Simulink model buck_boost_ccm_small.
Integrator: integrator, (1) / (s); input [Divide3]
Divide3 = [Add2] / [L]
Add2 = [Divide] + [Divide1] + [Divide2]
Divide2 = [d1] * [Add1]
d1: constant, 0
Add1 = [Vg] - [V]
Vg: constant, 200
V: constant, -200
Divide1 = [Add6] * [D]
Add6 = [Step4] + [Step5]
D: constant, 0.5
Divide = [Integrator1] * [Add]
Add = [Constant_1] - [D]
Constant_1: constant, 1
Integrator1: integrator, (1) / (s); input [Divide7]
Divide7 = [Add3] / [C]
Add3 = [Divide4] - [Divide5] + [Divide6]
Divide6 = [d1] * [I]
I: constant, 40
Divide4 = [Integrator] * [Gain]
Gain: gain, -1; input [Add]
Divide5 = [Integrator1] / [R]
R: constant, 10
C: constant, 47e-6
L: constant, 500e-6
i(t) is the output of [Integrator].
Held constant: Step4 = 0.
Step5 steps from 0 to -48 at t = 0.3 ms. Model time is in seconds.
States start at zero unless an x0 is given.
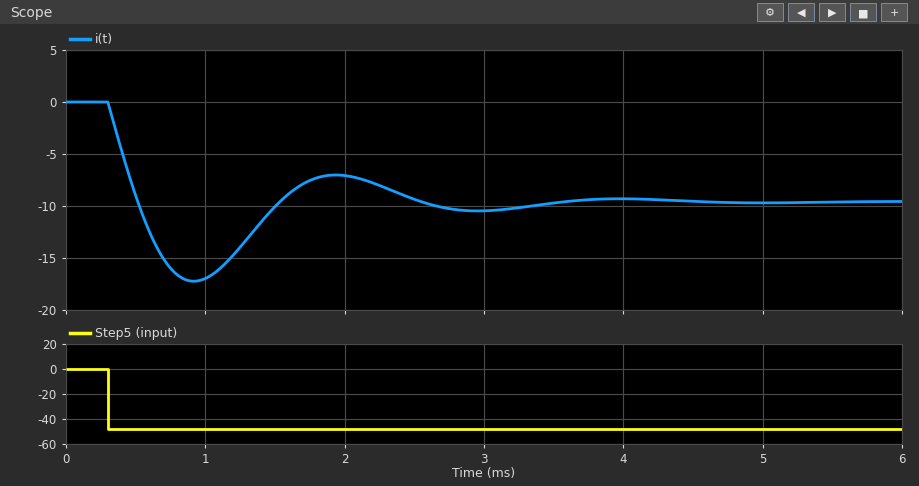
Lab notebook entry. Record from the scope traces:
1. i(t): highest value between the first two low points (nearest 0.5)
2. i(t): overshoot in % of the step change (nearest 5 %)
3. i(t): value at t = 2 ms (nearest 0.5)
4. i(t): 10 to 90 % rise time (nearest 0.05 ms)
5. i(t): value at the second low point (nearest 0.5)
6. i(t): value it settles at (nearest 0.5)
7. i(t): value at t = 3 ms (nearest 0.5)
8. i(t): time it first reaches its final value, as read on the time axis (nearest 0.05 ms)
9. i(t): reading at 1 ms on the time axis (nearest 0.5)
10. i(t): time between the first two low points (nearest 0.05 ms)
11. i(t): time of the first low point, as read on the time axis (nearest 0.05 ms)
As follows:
-7.0
80 %
-7.0
0.15 ms
-10.5
-9.5
-10.5
0.50 ms
-17.0
2.05 ms
0.90 ms
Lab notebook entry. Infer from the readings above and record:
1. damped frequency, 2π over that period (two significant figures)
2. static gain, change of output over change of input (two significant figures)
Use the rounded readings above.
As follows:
3.1 rad/ms
0.20
